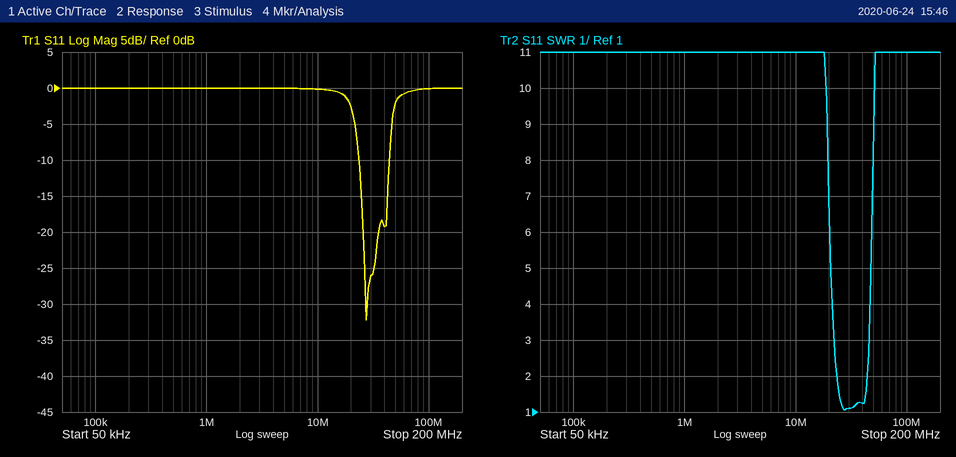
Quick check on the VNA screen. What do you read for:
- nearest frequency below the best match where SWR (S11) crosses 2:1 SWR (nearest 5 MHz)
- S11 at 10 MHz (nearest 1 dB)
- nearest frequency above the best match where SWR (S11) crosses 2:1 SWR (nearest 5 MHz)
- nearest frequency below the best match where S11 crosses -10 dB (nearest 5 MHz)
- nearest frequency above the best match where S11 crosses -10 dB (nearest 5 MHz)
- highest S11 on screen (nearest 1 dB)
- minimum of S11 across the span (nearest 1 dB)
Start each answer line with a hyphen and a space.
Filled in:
- 25 MHz
- 0 dB
- 45 MHz
- 25 MHz
- 45 MHz
- 0 dB
- -32 dB
